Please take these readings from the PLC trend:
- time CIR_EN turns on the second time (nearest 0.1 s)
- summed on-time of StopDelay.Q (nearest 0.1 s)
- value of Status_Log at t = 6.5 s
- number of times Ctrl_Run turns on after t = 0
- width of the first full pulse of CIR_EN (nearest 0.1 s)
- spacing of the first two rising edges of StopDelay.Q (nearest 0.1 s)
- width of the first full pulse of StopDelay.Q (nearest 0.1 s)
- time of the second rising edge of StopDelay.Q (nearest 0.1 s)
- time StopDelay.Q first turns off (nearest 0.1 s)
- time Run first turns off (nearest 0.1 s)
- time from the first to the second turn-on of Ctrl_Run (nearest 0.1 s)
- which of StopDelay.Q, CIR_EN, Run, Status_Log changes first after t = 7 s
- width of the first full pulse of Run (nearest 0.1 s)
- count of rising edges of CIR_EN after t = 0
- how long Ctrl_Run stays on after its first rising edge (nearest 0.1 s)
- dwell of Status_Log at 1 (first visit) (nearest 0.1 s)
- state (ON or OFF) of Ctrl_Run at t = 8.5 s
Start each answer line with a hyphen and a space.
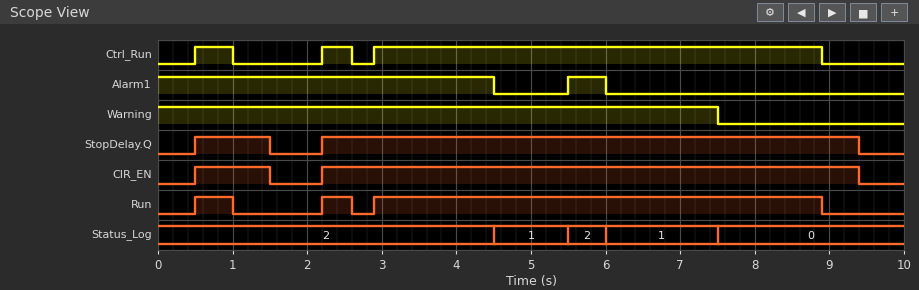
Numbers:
- 2.2 s
- 8.2 s
- 1
- 3
- 1.0 s
- 1.7 s
- 1.0 s
- 2.2 s
- 1.5 s
- 1.0 s
- 1.7 s
- Status_Log
- 0.5 s
- 2
- 0.5 s
- 1.0 s
- ON
